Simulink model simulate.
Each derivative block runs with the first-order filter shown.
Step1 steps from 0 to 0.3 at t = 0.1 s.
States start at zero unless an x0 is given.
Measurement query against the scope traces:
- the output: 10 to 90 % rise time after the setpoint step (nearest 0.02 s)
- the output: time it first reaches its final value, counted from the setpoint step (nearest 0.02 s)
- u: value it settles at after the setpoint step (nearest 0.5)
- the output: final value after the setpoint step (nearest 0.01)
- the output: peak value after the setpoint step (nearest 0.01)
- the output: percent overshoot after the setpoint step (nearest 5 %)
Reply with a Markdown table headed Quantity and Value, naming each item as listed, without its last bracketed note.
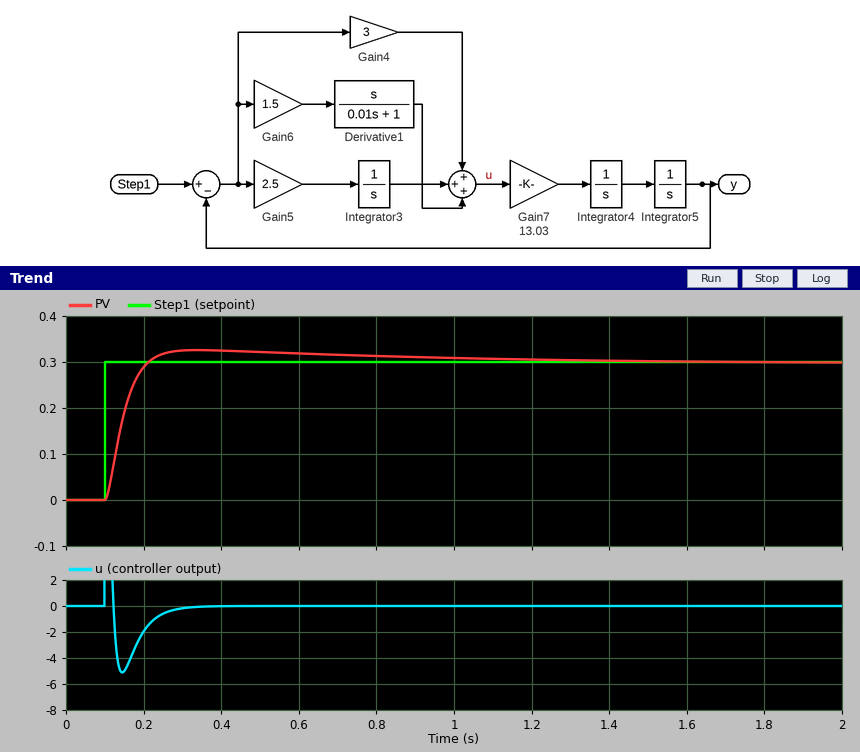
| Quantity | Value |
|---|---|
| the output: 10 to 90 % rise time after the setpoint step | 0.08 s |
| the output: time it first reaches its final value, counted from the setpoint step | 0.12 s |
| u: value it settles at after the setpoint step | 0.0 |
| the output: final value after the setpoint step | 0.30 |
| the output: peak value after the setpoint step | 0.33 |
| the output: percent overshoot after the setpoint step | 10 % |
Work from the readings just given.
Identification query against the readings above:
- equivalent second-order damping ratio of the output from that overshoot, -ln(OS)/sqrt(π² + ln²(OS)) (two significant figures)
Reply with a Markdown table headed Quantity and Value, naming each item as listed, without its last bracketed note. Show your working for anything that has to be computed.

| Quantity | Value |
|---|---|
| equivalent second-order damping ratio of the output from that overshoot, -ln(OS)/sqrt(π² + ln²(OS)) | ln(0.1) = -2.303; 2.303 / sqrt(9.870 + 5.302) = 0.59 |
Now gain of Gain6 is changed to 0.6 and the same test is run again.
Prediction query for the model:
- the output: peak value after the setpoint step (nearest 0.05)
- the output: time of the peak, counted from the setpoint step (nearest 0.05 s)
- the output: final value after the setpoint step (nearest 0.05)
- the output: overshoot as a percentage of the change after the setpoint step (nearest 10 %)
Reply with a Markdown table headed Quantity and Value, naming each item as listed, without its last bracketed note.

| Quantity | Value |
|---|---|
| the output: peak value after the setpoint step | 0.40 |
| the output: time of the peak, counted from the setpoint step | 0.35 s |
| the output: final value after the setpoint step | 0.30 |
| the output: overshoot as a percentage of the change after the setpoint step | 30 % |
